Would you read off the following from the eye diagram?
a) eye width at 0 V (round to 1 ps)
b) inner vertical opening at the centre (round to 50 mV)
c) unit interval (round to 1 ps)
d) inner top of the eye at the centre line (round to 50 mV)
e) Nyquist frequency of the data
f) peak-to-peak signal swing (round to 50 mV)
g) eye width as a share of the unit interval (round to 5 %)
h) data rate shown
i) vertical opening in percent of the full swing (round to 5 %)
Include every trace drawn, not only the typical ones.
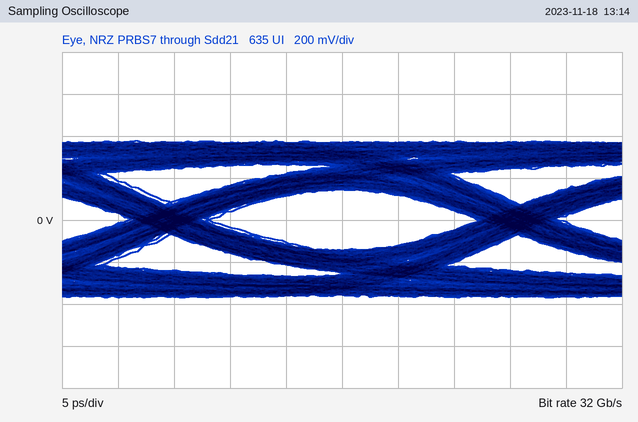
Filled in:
24 ps
300 mV
31 ps
150 mV
16 GHz
750 mV
75 %
32 Gb/s
40 %
